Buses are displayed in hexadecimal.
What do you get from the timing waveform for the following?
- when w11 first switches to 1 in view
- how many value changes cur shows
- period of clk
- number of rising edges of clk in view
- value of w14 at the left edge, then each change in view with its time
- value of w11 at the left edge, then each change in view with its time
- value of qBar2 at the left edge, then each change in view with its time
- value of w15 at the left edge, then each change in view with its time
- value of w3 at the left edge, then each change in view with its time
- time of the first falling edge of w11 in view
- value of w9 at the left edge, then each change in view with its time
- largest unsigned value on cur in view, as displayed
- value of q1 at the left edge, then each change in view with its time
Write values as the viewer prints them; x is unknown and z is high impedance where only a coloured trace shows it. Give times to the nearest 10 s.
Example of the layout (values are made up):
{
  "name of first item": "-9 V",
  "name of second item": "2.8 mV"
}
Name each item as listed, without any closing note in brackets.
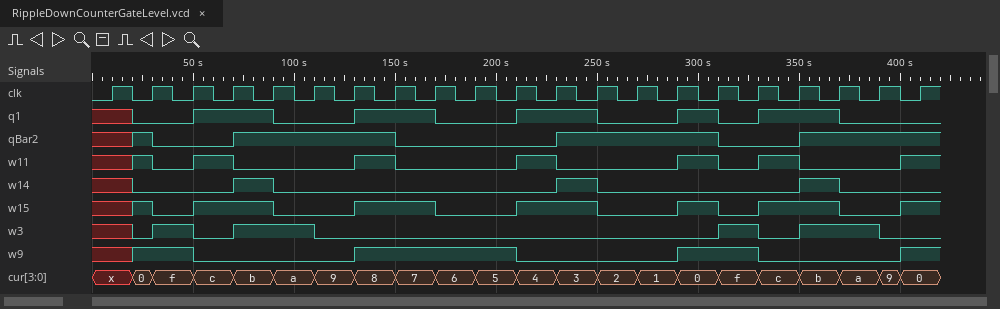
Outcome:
{
  "when w11 first switches to 1 in view": "20 s",
  "how many value changes cur shows": "21",
  "period of clk": "20 s",
  "number of rising edges of clk in view": "21",
  "value of w14 at the left edge, then each change in view with its time": "x, 0 at 20 s, 1 at 70 s, 0 at 90 s, 1 at 230 s, 0 at 250 s, 1 at 350 s, 0 at 370 s",
  "value of w11 at the left edge, then each change in view with its time": "x, 1 at 20 s, 0 at 30 s, 1 at 50 s, 0 at 70 s, 1 at 130 s, 0 at 150 s, 1 at 210 s, 0 at 230 s, 1 at 290 s, 0 at 310 s, 1 at 330 s, 0 at 350 s, 1 at 400 s",
  "value of qBar2 at the left edge, then each change in view with its time": "x, 1 at 20 s, 0 at 30 s, 1 at 70 s, 0 at 150 s, 1 at 230 s, 0 at 310 s, 1 at 350 s",
  "value of w15 at the left edge, then each change in view with its time": "x, 1 at 20 s, 0 at 30 s, 1 at 50 s, 0 at 90 s, 1 at 130 s, 0 at 170 s, 1 at 210 s, 0 at 250 s, 1 at 290 s, 0 at 310 s, 1 at 330 s, 0 at 370 s, 1 at 400 s",
  "value of w3 at the left edge, then each change in view with its time": "x, 0 at 20 s, 1 at 30 s, 0 at 50 s, 1 at 70 s, 0 at 110 s, 1 at 310 s, 0 at 330 s, 1 at 350 s, 0 at 390 s",
  "time of the first falling edge of w11 in view": "30 s",
  "value of w9 at the left edge, then each change in view with its time": "x, 1 at 20 s, 0 at 50 s, 1 at 130 s, 0 at 210 s, 1 at 290 s, 0 at 330 s, 1 at 400 s",
  "largest unsigned value on cur in view, as displayed": "f",
  "value of q1 at the left edge, then each change in view with its time": "x, 0 at 20 s, 1 at 50 s, 0 at 90 s, 1 at 130 s, 0 at 170 s, 1 at 210 s, 0 at 250 s, 1 at 290 s, 0 at 310 s, 1 at 330 s, 0 at 370 s"
}
